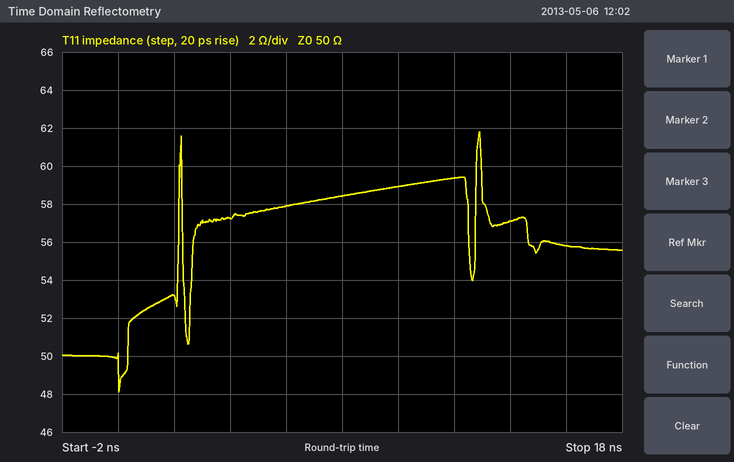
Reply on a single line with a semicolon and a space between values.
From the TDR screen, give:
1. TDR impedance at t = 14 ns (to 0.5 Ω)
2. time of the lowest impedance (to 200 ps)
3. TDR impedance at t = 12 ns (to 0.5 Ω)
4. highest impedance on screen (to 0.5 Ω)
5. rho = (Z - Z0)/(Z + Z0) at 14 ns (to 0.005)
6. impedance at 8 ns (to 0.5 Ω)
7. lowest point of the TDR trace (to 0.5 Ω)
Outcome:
57.0 Ω; 0.0 ns; 59.5 Ω; 62.0 Ω; +0.065; 58.5 Ω; 48.0 Ω
